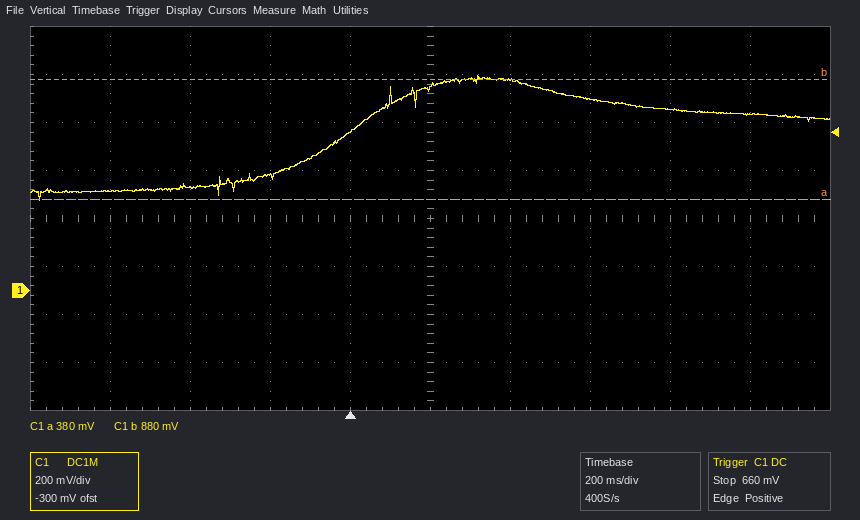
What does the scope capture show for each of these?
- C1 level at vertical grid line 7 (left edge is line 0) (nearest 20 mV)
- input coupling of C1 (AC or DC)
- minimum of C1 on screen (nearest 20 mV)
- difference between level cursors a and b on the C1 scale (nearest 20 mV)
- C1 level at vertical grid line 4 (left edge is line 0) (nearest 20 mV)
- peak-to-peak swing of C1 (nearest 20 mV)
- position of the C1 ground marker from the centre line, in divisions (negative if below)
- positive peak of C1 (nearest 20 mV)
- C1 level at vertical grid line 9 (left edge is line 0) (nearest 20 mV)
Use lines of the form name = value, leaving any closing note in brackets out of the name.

C1 level at vertical grid line 7 (left edge is line 0) = 800 mV
input coupling of C1 = DC
minimum of C1 on screen = 380 mV
difference between level cursors a and b on the C1 scale = 500 mV
C1 level at vertical grid line 4 (left edge is line 0) = 660 mV
peak-to-peak swing of C1 = 520 mV
position of the C1 ground marker from the centre line, in divisions = -1.5 div
positive peak of C1 = 900 mV
C1 level at vertical grid line 9 (left edge is line 0) = 740 mV
